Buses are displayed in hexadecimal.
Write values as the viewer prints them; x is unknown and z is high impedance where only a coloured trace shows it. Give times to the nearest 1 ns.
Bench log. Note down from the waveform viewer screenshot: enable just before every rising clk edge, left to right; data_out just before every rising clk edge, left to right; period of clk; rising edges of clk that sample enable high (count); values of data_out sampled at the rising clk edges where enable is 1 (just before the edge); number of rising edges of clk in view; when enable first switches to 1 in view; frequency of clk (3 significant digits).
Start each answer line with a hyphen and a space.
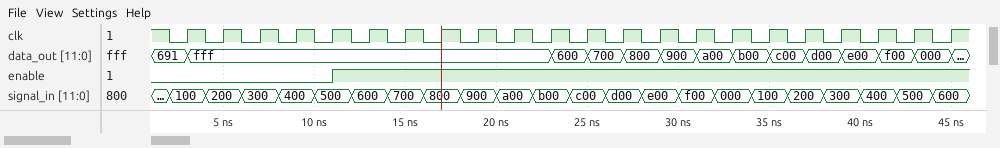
- 0 0 0 0 0 1 1 1 1 1 1 1 1 1 1 1 1 1 1 1 1 1
- 691, fff, fff, fff, fff, fff, fff, fff, fff, fff, fff, 600, 700, 800, 900, a00, b00, c00, d00, e00, f00, 000
- 2 ns
- 17
- fff, fff, fff, fff, fff, fff, 600, 700, 800, 900, a00, b00, c00, d00, e00, f00, 000
- 22
- 11 ns
- 500 MHz
